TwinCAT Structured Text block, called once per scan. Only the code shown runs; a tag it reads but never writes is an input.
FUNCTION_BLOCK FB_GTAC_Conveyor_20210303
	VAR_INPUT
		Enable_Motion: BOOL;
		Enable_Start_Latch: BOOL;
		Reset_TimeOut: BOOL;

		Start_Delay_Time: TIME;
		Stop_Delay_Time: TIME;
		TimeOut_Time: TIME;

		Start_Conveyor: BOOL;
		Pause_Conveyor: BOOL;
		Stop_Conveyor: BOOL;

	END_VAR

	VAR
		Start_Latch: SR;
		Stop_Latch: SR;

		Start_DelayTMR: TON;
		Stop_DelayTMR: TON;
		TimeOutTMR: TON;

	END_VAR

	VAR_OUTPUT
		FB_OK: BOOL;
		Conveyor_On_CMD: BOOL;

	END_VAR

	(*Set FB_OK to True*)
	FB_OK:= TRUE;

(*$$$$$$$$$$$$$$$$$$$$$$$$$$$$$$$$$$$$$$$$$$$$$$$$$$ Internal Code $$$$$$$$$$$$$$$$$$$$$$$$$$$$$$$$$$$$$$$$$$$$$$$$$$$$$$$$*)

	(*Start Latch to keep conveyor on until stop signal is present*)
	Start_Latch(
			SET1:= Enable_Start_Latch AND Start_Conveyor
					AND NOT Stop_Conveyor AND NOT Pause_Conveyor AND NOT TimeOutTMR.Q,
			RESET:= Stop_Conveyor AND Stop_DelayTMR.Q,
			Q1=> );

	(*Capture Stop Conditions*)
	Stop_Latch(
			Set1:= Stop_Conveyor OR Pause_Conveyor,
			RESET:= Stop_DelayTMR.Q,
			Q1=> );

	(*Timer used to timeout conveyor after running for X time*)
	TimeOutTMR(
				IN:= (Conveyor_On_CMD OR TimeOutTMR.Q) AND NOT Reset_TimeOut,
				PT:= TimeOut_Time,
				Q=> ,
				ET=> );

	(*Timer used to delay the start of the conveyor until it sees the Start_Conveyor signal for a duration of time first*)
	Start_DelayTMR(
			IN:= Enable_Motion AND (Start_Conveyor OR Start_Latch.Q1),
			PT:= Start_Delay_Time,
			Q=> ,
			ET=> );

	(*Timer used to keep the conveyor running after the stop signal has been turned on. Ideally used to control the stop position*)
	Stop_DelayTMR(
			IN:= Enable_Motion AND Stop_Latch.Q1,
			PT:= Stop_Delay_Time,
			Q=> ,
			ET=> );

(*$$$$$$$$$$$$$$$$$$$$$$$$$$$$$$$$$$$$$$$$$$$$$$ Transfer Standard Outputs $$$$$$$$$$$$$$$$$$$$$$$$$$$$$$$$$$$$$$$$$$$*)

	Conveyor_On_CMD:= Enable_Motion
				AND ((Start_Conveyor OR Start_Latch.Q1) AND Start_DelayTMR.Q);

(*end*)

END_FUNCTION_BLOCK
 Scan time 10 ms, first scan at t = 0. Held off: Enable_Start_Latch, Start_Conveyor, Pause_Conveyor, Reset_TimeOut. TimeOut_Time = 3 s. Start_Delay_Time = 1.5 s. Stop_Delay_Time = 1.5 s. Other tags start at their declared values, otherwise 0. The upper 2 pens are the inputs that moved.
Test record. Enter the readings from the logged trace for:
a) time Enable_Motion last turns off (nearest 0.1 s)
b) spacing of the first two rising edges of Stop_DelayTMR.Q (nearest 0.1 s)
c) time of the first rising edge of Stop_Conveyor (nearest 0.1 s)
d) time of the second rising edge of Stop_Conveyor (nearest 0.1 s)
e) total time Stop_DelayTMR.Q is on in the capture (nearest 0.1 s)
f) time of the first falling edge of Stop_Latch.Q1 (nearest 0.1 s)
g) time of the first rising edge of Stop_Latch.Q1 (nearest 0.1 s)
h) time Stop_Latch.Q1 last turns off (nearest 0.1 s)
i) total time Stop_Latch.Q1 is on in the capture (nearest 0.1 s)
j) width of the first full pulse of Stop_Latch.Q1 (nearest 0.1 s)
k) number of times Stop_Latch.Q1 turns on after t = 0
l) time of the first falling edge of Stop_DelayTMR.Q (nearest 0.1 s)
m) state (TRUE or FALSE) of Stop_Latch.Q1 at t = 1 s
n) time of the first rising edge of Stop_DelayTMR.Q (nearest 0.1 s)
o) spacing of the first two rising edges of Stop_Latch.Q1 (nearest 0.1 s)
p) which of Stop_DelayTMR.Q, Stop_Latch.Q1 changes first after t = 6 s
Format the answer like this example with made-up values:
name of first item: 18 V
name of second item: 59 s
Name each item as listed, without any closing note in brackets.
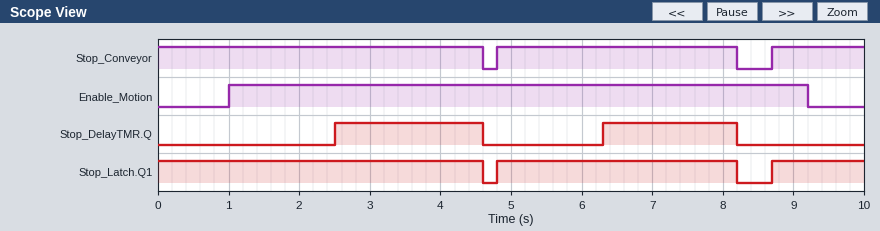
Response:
time Enable_Motion last turns off: 9.2 s
spacing of the first two rising edges of Stop_DelayTMR.Q: 3.8 s
time of the first rising edge of Stop_Conveyor: 4.8 s
time of the second rising edge of Stop_Conveyor: 8.7 s
total time Stop_DelayTMR.Q is on in the capture: 4.0 s
time of the first falling edge of Stop_Latch.Q1: 4.6 s
time of the first rising edge of Stop_Latch.Q1: 4.8 s
time Stop_Latch.Q1 last turns off: 8.2 s
total time Stop_Latch.Q1 is on in the capture: 9.3 s
width of the first full pulse of Stop_Latch.Q1: 3.4 s
number of times Stop_Latch.Q1 turns on after t = 0: 2
time of the first falling edge of Stop_DelayTMR.Q: 4.6 s
state (TRUE or FALSE) of Stop_Latch.Q1 at t = 1 s: TRUE
time of the first rising edge of Stop_DelayTMR.Q: 2.5 s
spacing of the first two rising edges of Stop_Latch.Q1: 3.9 s
which of Stop_DelayTMR.Q, Stop_Latch.Q1 changes first after t = 6 s: Stop_DelayTMR.Q
